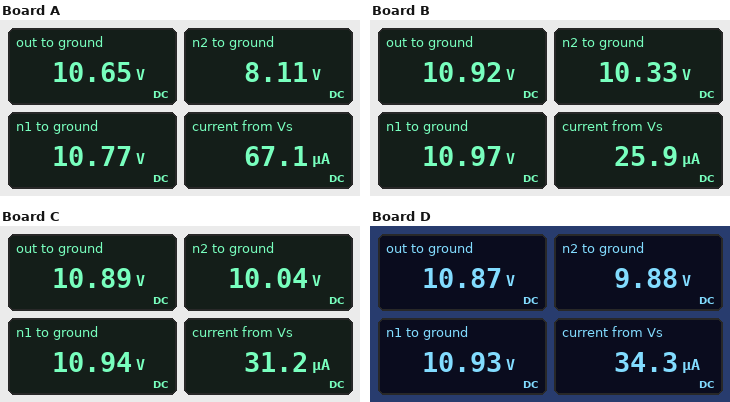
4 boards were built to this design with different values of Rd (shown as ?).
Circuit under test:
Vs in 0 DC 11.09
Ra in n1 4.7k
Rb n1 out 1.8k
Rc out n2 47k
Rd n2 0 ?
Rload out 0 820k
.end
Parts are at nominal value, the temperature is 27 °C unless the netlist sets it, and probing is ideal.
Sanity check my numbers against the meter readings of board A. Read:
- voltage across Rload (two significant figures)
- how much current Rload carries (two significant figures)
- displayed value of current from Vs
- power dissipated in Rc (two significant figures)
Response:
11 V
13 µA
67.1 µA
140 µW
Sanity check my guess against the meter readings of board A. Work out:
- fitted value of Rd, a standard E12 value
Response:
150 kΩ
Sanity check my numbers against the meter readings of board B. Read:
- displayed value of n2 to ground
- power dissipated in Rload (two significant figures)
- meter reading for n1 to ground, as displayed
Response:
10.33 V
150 µW
10.97 V
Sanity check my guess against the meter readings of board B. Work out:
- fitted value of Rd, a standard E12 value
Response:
820 kΩ
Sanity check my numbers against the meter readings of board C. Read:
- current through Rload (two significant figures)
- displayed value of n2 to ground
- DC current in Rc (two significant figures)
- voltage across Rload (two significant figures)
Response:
13 µA
10.04 V
18 µA
11 V
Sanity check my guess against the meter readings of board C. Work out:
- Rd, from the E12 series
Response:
560 kΩ
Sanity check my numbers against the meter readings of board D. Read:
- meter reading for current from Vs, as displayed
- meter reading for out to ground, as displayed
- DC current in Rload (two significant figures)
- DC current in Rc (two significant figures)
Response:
34.3 µA
10.87 V
13 µA
21 µA
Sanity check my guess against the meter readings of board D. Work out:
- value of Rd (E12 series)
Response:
470 kΩ
